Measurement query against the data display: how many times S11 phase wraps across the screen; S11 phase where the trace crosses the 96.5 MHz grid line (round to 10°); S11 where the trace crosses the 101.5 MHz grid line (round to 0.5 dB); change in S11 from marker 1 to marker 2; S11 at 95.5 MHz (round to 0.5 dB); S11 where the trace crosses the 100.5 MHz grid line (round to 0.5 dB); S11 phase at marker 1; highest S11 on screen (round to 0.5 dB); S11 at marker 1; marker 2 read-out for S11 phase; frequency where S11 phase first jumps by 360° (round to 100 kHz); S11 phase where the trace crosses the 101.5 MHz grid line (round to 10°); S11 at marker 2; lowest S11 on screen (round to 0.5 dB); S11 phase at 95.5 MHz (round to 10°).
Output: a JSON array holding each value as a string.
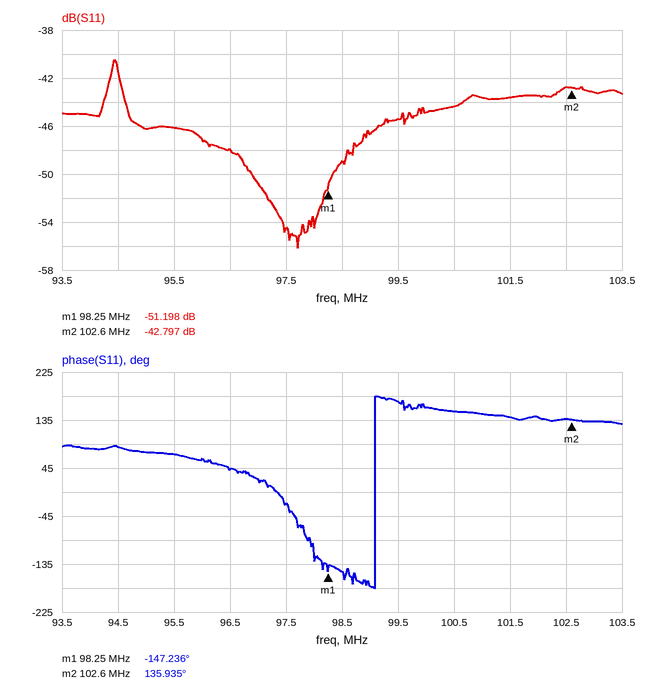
["1", "40°", "-43.5 dB", "8.401 dB", "-46.0 dB", "-44.5 dB", "-147.236°", "-40.5 dB", "-51.198 dB", "135.935°", "99.1 MHz", "140°", "-42.797 dB", "-56.0 dB", "70°"]
